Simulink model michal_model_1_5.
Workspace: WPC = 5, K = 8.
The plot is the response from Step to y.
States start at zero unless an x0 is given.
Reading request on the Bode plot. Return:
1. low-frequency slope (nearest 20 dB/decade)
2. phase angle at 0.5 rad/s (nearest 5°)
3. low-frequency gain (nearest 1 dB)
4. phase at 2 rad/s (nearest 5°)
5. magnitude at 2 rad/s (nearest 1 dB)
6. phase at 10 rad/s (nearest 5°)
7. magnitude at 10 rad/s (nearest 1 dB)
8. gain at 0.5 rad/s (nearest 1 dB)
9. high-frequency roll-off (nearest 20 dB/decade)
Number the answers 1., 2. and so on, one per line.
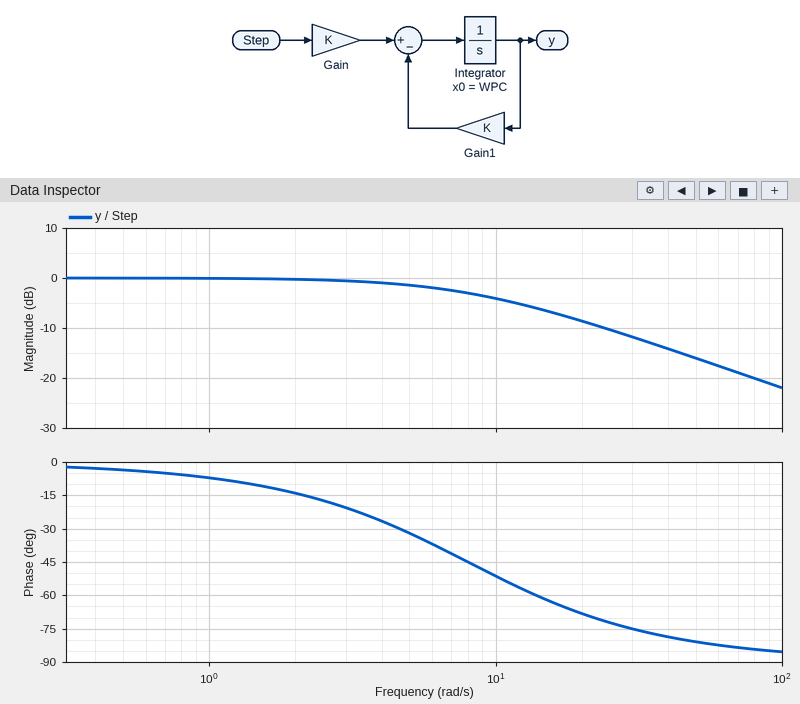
1. 0 dB/decade
2. -5°
3. 0 dB
4. -15°
5. 0 dB
6. -50°
7. -4 dB
8. 0 dB
9. -20 dB/decade
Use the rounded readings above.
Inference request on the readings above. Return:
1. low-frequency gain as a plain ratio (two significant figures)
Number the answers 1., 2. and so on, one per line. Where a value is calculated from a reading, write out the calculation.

1. 10^(0 / 20) = 1.0
